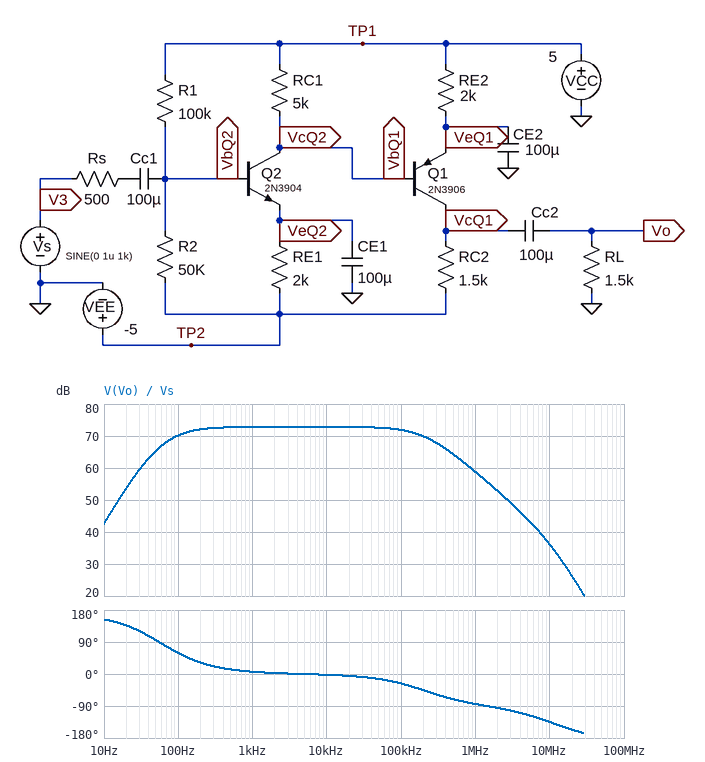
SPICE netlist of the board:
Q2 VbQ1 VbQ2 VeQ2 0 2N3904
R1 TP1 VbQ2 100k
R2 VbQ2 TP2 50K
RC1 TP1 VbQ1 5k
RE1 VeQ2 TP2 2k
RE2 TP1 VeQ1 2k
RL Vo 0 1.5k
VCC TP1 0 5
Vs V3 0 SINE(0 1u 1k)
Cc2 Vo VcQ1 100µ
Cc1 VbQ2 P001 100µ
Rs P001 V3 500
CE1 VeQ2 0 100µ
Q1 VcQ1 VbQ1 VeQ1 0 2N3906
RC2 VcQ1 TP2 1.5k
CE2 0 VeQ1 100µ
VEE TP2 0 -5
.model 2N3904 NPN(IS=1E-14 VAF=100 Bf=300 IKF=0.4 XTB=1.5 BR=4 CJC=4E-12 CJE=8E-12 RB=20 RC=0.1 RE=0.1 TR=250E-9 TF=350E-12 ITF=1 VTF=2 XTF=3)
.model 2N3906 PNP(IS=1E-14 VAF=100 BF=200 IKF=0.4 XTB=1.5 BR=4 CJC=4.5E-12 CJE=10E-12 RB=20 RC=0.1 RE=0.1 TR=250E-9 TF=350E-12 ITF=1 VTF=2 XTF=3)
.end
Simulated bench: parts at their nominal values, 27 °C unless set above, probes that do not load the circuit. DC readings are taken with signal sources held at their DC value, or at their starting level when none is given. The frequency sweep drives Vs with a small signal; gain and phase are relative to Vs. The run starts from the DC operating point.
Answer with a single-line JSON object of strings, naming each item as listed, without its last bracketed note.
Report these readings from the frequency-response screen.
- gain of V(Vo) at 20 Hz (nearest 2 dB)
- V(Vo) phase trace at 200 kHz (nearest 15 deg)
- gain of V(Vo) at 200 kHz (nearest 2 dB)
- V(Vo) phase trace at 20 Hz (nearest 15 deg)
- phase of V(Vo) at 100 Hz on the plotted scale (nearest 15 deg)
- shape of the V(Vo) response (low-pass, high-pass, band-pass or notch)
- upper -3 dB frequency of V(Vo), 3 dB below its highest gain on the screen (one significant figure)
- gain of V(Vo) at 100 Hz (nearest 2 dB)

{"gain of V(Vo) at 20 Hz": "54 dB", "V(Vo) phase trace at 200 kHz": "-45 deg", "gain of V(Vo) at 200 kHz": "70 dB", "V(Vo) phase trace at 20 Hz": "135 deg", "phase of V(Vo) at 100 Hz on the plotted scale": "60 deg", "shape of the V(Vo) response": "band-pass", "upper -3 dB frequency of V(Vo), 3 dB below its highest gain on the screen": "200 kHz", "gain of V(Vo) at 100 Hz": "70 dB"}
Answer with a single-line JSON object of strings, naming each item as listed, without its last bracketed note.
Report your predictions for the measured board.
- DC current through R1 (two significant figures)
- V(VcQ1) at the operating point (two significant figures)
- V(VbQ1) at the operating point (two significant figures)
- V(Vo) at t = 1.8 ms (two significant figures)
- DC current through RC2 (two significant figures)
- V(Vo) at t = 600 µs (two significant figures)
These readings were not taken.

{"DC current through R1": "68 µA", "V(VcQ1) at the operating point": "-850 mV", "V(VbQ1) at the operating point": "-1.2 V", "V(Vo) at t = 1.8 ms": "-4.2 mV", "DC current through RC2": "2.8 mA", "V(Vo) at t = 600 µs": "-3.3 mV"}
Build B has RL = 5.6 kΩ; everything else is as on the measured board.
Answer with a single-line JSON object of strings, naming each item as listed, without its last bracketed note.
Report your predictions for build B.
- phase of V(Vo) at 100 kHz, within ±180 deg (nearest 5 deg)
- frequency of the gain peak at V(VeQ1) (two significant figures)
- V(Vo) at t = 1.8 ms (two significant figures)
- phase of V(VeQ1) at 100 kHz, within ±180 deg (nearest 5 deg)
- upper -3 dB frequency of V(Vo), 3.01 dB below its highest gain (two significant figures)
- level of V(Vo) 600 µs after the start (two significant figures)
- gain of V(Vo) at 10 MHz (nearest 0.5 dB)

{"phase of V(Vo) at 100 kHz, within ±180 deg": "-35 deg", "frequency of the gain peak at V(VeQ1)": "55 Hz", "V(Vo) at t = 1.8 ms": "-6.4 mV", "phase of V(VeQ1) at 100 kHz, within ±180 deg": "55 deg", "upper -3 dB frequency of V(Vo), 3.01 dB below its highest gain": "140 kHz", "level of V(Vo) 600 µs after the start": "-5.0 mV", "gain of V(Vo) at 10 MHz": "36.5 dB"}
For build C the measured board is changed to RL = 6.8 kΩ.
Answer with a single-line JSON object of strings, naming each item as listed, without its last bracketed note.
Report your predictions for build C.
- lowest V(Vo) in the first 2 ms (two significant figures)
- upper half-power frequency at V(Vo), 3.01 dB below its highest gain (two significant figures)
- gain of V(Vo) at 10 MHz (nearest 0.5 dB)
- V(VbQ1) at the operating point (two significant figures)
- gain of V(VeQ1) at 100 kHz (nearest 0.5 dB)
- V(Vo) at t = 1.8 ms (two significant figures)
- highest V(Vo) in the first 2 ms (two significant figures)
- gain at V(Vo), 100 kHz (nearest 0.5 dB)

{"lowest V(Vo) in the first 2 ms": "-7.5 mV", "upper half-power frequency at V(Vo), 3.01 dB below its highest gain": "140 kHz", "gain of V(Vo) at 10 MHz": "36.5 dB", "V(VbQ1) at the operating point": "-1.2 V", "gain of V(VeQ1) at 100 kHz": "-22.5 dB", "V(Vo) at t = 1.8 ms": "-6.6 mV", "highest V(Vo) in the first 2 ms": "6.5 mV", "gain at V(Vo), 100 kHz": "75.0 dB"}
